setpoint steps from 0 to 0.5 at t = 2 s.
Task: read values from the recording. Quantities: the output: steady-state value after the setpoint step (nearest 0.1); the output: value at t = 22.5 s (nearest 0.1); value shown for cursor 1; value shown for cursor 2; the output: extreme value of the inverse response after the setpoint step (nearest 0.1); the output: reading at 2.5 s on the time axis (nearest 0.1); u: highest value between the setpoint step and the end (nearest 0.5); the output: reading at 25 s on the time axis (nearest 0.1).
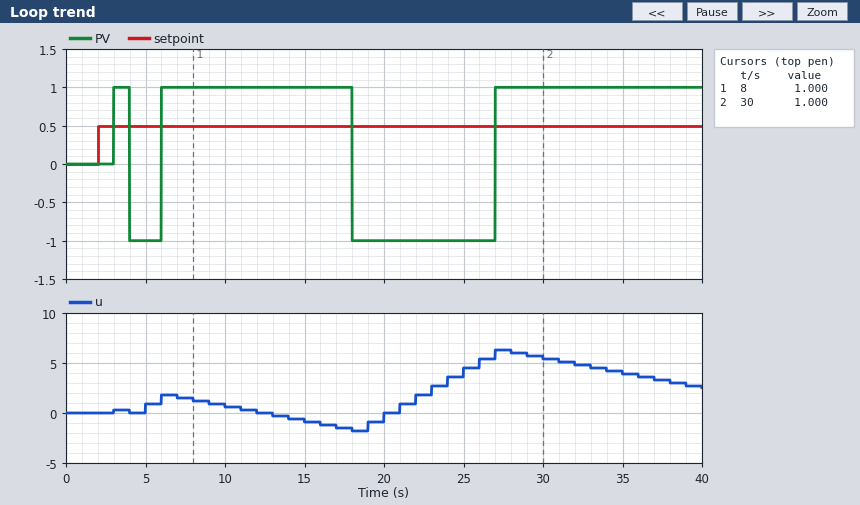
1.0
-1.0
1.000
1.000
-1.0
0.0
6.5
-1.0
